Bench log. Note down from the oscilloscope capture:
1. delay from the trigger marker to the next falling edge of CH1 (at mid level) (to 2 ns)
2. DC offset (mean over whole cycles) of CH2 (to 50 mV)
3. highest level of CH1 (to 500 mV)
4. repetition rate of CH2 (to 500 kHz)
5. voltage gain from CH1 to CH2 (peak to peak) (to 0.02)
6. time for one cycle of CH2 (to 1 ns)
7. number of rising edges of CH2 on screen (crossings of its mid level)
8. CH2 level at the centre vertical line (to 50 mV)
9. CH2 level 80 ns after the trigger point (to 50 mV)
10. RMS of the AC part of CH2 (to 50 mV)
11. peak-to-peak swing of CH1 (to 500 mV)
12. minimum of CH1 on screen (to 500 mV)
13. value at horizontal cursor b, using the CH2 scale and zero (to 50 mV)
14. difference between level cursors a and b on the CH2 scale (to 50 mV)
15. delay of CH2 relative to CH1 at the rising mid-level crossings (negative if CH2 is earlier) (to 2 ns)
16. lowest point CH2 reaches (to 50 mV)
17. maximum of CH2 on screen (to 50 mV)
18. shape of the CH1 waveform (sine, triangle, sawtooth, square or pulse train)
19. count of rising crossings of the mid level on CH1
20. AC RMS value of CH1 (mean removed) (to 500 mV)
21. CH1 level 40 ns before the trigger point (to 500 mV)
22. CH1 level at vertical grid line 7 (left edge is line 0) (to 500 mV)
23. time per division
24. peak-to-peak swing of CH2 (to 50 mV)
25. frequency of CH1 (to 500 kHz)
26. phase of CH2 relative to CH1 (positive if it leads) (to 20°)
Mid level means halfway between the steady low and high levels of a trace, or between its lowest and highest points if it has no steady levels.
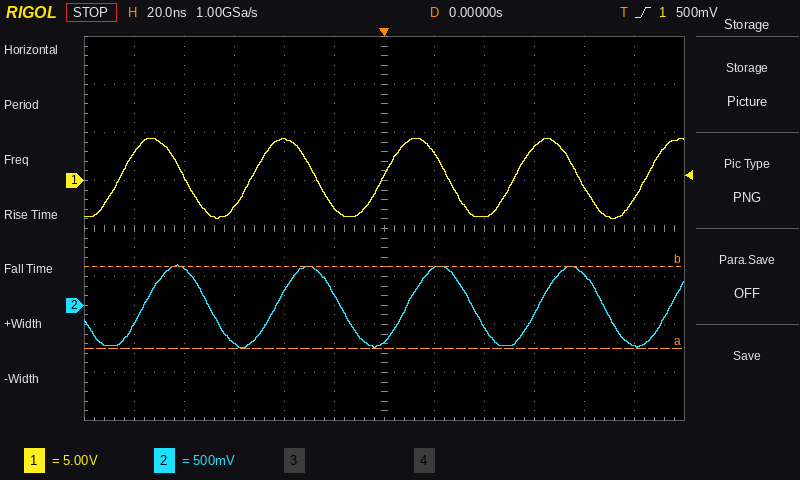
26 ns
0 mV
4.5 V
19.0 MHz
0.10
53 ns
5
-400 mV
300 mV
300 mV
8.5 V
-4.0 V
400 mV
850 mV
+10 ns
-450 mV
400 mV
sine
5
3.0 V
4.5 V
3.0 V
20 ns
850 mV
19.0 MHz
-60°
